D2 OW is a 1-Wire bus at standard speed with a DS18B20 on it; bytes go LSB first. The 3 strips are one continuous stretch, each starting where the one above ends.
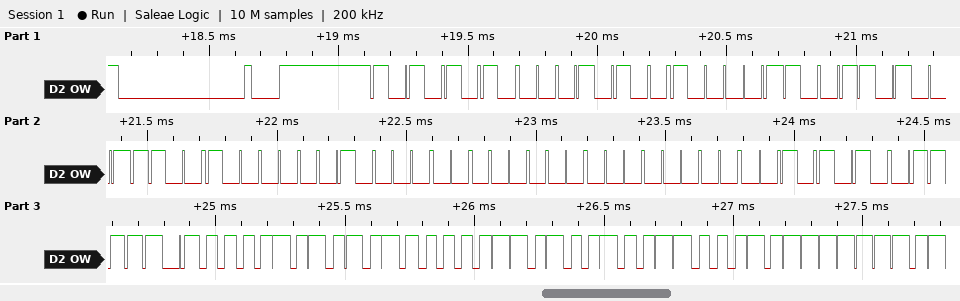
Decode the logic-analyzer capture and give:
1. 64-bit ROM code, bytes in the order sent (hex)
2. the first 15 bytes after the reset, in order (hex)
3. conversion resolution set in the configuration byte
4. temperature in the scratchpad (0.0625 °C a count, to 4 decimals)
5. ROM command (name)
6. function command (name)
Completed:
28 61 96 13 08 00 00 54
55 28 61 96 13 08 00 00 54 BE 50 05 4B 46 7F
12 bits
85.0000 °C
Match ROM
Read Scratchpad
